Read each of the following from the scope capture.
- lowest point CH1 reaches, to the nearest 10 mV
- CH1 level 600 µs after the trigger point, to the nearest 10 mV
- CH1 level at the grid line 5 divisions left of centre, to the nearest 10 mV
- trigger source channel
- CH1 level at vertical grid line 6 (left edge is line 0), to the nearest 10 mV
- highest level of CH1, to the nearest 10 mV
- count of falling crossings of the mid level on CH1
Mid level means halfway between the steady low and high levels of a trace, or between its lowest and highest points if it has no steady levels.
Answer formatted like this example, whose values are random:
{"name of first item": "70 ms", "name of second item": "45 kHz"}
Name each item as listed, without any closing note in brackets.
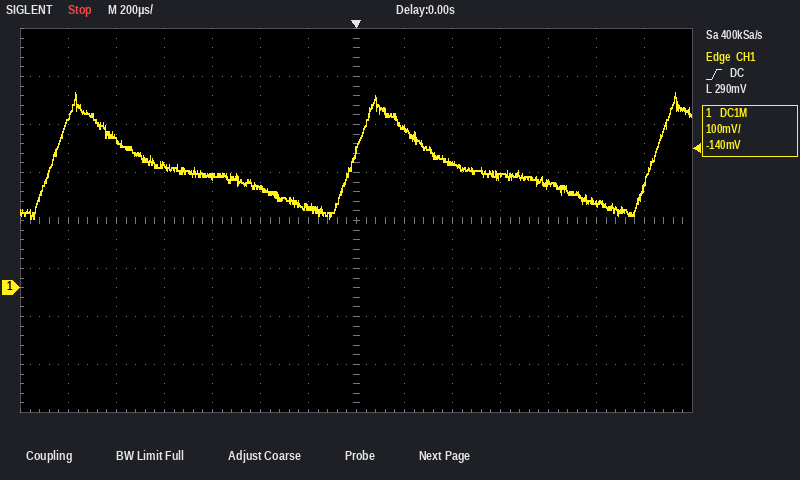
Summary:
{"lowest point CH1 reaches, to the nearest 10 mV": "140 mV", "CH1 level 600 µs after the trigger point, to the nearest 10 mV": "230 mV", "CH1 level at the grid line 5 divisions left of centre, to the nearest 10 mV": "310 mV", "trigger source channel": "CH1", "CH1 level at vertical grid line 6 (left edge is line 0), to the nearest 10 mV": "170 mV", "highest level of CH1, to the nearest 10 mV": "410 mV", "count of falling crossings of the mid level on CH1": "2"}
